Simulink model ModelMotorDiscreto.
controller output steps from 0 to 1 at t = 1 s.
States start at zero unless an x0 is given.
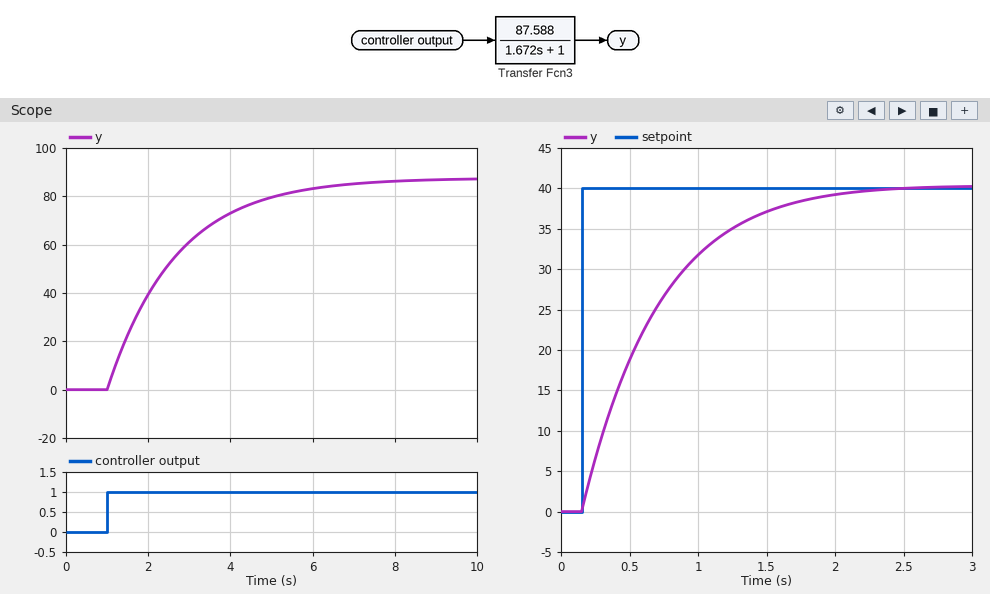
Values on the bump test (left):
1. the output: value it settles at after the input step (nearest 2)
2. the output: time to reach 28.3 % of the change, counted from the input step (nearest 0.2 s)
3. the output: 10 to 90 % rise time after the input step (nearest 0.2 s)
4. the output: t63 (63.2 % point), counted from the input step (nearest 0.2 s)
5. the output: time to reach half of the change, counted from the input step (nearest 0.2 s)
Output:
88
0.6 s
3.6 s
1.6 s
1.2 s
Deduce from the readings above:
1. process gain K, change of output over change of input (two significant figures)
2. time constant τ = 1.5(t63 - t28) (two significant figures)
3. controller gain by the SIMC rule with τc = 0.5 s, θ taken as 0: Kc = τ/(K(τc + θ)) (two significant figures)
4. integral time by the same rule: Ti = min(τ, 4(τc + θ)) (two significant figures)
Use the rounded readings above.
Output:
88
1.5 s
0.034
1.5 s
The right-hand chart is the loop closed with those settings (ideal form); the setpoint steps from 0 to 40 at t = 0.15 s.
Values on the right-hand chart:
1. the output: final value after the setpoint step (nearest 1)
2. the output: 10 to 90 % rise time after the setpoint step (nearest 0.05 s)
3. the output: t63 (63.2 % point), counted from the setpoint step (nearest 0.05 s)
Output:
40
1.15 s
0.55 s
